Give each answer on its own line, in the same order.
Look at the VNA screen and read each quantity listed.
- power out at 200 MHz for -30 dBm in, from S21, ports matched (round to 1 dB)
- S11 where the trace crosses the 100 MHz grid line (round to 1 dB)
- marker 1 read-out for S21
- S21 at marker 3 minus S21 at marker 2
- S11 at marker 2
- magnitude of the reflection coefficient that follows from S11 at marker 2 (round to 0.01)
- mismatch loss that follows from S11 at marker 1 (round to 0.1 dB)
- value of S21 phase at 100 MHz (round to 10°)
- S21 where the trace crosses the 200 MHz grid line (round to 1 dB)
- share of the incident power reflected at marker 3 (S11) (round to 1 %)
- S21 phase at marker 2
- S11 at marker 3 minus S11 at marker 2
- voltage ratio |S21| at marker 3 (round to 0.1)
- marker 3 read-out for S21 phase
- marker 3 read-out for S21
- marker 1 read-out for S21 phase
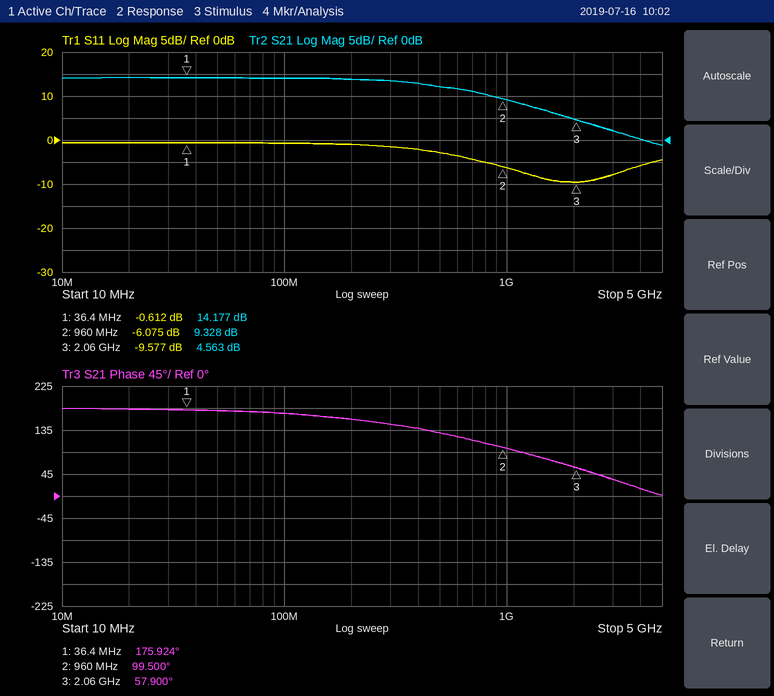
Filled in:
-16 dBm
-1 dB
14.177 dB
-4.765 dB
-6.075 dB
0.50
8.8 dB
170°
14 dB
11 %
99.500°
-3.502 dB
1.7
57.900°
4.563 dB
175.924°
